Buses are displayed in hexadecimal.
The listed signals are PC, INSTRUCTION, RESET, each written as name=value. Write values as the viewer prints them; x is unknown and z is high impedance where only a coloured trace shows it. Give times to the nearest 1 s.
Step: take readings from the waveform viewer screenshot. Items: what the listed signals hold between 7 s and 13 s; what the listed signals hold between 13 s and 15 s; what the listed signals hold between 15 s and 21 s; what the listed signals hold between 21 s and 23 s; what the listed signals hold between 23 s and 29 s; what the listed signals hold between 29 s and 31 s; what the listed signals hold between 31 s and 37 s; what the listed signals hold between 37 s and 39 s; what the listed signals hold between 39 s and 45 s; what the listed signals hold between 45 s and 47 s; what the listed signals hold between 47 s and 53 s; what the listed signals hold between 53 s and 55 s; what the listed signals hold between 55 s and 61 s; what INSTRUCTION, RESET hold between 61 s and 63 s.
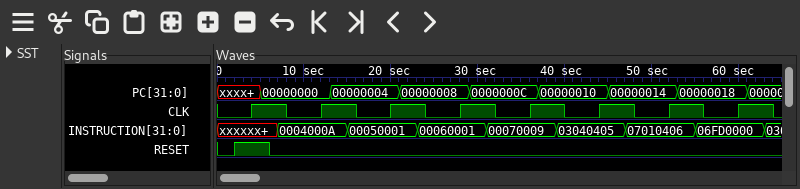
PC=00000000, INSTRUCTION=0004000A, RESET=0
PC=00000004, INSTRUCTION=0004000A, RESET=0
PC=00000004, INSTRUCTION=00050001, RESET=0
PC=00000008, INSTRUCTION=00050001, RESET=0
PC=00000008, INSTRUCTION=00060001, RESET=0
PC=0000000C, INSTRUCTION=00060001, RESET=0
PC=0000000C, INSTRUCTION=00070009, RESET=0
PC=00000010, INSTRUCTION=00070009, RESET=0
PC=00000010, INSTRUCTION=03040405, RESET=0
PC=00000014, INSTRUCTION=03040405, RESET=0
PC=00000014, INSTRUCTION=07010406, RESET=0
PC=00000018, INSTRUCTION=07010406, RESET=0
PC=00000018, INSTRUCTION=06FD0000, RESET=0
INSTRUCTION=06FD0000, RESET=0
